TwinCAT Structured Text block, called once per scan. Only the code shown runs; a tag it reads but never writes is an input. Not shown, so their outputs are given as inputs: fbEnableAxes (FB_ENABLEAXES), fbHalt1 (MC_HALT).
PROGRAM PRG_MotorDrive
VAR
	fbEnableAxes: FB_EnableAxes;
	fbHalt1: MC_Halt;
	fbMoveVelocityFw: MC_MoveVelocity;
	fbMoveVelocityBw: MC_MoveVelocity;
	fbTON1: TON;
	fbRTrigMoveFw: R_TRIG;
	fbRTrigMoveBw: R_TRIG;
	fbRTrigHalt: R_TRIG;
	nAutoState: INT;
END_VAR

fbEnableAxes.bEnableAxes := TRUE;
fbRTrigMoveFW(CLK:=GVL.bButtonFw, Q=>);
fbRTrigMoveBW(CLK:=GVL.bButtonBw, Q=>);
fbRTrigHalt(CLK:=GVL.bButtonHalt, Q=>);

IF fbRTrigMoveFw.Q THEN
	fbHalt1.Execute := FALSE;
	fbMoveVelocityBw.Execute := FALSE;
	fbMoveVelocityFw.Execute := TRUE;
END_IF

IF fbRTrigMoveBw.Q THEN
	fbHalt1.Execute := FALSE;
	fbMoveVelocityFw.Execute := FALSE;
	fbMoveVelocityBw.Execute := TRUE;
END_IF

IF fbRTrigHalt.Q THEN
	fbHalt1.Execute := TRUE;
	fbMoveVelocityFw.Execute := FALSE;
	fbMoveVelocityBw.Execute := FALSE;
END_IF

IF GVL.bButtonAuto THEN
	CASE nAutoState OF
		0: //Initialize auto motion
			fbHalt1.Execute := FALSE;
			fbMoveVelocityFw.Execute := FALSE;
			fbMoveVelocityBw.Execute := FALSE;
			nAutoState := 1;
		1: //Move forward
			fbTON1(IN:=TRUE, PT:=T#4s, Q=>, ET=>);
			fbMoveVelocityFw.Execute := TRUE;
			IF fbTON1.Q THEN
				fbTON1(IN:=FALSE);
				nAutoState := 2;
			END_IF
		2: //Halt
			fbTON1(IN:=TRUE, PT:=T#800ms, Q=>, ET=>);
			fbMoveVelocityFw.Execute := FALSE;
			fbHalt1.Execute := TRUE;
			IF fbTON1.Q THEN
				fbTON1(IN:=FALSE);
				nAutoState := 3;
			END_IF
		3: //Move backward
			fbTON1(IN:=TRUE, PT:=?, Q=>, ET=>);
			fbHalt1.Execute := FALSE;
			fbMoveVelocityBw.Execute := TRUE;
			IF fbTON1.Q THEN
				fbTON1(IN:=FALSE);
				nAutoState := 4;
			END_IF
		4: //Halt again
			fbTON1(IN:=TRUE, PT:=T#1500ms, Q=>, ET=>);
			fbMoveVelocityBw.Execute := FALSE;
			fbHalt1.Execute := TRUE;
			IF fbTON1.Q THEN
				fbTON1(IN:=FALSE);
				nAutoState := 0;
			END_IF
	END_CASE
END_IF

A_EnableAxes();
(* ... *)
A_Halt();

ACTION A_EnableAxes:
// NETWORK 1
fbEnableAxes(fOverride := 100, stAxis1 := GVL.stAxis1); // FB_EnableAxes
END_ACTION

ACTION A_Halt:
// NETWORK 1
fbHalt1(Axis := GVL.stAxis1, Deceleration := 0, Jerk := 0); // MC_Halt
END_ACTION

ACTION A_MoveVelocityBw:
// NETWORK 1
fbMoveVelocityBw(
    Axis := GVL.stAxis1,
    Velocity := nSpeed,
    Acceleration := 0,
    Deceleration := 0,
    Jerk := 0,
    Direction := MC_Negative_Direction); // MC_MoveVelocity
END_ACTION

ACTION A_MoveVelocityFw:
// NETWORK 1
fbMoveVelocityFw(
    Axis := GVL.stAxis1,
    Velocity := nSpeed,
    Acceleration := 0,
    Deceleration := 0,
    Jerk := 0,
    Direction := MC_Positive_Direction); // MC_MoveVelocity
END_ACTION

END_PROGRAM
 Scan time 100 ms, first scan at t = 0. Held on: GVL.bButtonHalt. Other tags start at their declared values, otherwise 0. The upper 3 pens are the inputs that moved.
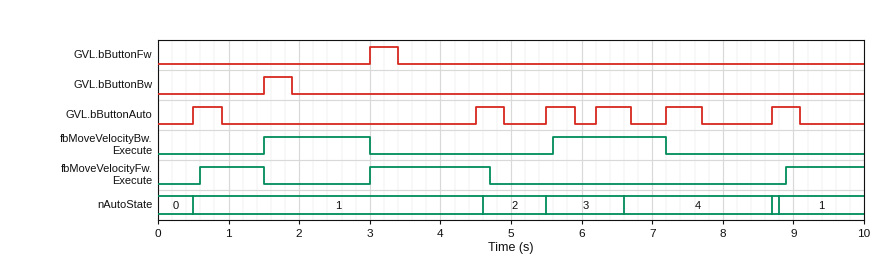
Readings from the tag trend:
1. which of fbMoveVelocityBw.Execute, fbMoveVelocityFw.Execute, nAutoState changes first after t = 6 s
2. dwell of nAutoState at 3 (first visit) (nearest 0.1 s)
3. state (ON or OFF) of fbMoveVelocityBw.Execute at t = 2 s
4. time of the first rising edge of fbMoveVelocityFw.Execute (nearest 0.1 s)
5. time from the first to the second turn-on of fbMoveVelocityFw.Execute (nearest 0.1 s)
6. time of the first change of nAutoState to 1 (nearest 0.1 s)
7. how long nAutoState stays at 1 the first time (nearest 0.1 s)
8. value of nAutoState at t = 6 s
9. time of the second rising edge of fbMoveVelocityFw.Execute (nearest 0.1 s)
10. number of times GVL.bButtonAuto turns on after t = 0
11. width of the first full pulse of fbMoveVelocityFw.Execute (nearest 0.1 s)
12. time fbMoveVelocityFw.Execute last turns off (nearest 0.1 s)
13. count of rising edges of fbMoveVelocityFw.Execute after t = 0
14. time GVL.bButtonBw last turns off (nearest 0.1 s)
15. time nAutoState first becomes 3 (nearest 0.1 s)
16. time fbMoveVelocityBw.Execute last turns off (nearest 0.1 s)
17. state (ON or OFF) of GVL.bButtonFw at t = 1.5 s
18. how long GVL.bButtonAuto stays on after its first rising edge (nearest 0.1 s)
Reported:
nAutoState
1.1 s
ON
0.6 s
2.4 s
0.5 s
4.1 s
3
3.0 s
6
0.9 s
4.7 s
3
1.9 s
5.5 s
7.2 s
OFF
0.4 s
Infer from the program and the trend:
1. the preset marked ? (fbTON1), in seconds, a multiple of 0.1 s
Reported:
1.0 s
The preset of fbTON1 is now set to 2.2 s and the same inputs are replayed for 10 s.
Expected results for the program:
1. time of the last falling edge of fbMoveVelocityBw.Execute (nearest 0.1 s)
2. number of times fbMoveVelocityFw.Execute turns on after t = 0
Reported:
8.8 s
2
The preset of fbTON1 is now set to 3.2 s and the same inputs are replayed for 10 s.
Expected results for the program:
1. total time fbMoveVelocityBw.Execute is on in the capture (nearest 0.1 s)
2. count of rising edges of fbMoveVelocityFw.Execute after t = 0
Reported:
4.8 s
2
